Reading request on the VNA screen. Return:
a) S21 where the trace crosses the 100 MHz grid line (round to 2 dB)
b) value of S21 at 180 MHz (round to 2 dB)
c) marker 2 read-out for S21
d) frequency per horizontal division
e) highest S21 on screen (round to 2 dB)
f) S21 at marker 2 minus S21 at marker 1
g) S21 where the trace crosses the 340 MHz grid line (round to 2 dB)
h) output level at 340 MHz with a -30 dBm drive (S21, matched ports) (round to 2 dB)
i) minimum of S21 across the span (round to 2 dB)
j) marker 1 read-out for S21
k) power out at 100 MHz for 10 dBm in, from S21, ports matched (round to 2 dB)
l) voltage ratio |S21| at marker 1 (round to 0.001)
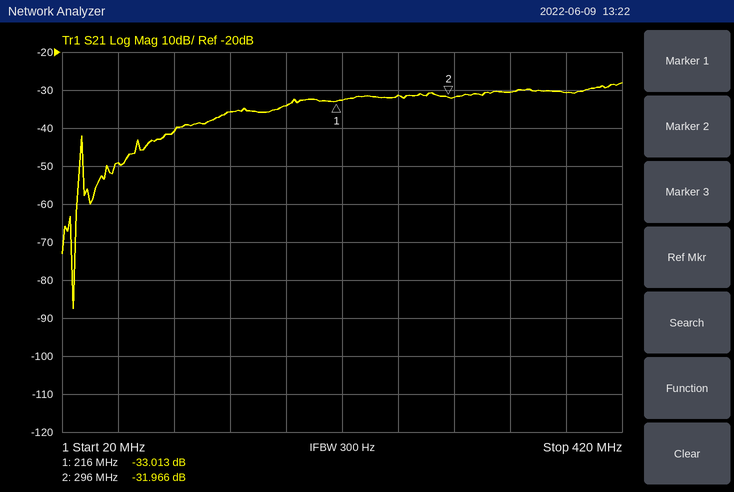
-40 dB
-34 dB
-31.966 dB
40 MHz
-28 dB
1.047 dB
-30 dB
-60 dBm
-88 dB
-33.013 dB
-30 dBm
0.022
